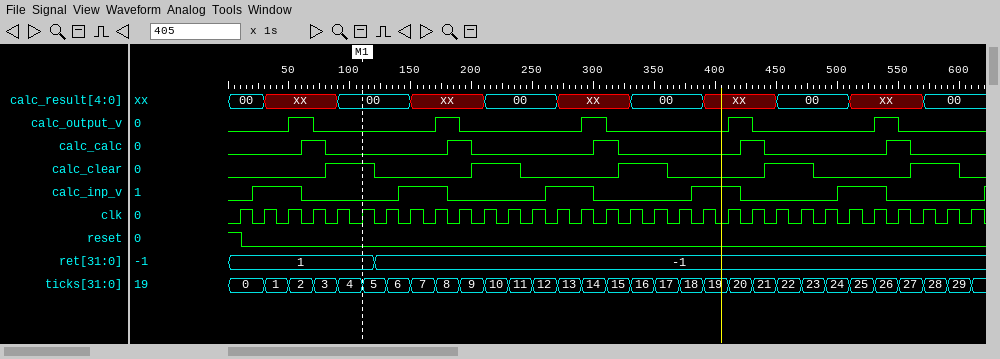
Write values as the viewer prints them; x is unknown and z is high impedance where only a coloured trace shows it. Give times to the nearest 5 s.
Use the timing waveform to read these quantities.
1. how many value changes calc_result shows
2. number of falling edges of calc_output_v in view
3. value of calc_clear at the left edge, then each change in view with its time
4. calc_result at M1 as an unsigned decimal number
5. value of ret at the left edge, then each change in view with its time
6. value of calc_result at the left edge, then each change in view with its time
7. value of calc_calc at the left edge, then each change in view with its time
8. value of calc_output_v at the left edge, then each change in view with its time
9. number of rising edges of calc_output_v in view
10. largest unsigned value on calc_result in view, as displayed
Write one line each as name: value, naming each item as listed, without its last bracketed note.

how many value changes calc_result shows: 10
number of falling edges of calc_output_v in view: 5
value of calc_clear at the left edge, then each change in view with its time: 0, 1 at 80 s, 0 at 120 s, 1 at 200 s, 0 at 240 s, 1 at 320 s, 0 at 360 s, 1 at 440 s, 0 at 480 s, 1 at 560 s, 0 at 600 s
calc_result at M1 as an unsigned decimal number: 0
value of ret at the left edge, then each change in view with its time: 1, -1 at 120 s
value of calc_result at the left edge, then each change in view with its time: 00, xx at 30 s, 00 at 90 s, xx at 150 s, 00 at 210 s, xx at 270 s, 00 at 330 s, xx at 390 s, 00 at 450 s, xx at 510 s, 00 at 570 s
value of calc_calc at the left edge, then each change in view with its time: 0, 1 at 60 s, 0 at 80 s, 1 at 180 s, 0 at 200 s, 1 at 300 s, 0 at 320 s, 1 at 420 s, 0 at 440 s, 1 at 540 s, 0 at 560 s
value of calc_output_v at the left edge, then each change in view with its time: 0, 1 at 50 s, 0 at 70 s, 1 at 170 s, 0 at 190 s, 1 at 290 s, 0 at 310 s, 1 at 410 s, 0 at 430 s, 1 at 530 s, 0 at 550 s
number of rising edges of calc_output_v in view: 5
largest unsigned value on calc_result in view, as displayed: 00
